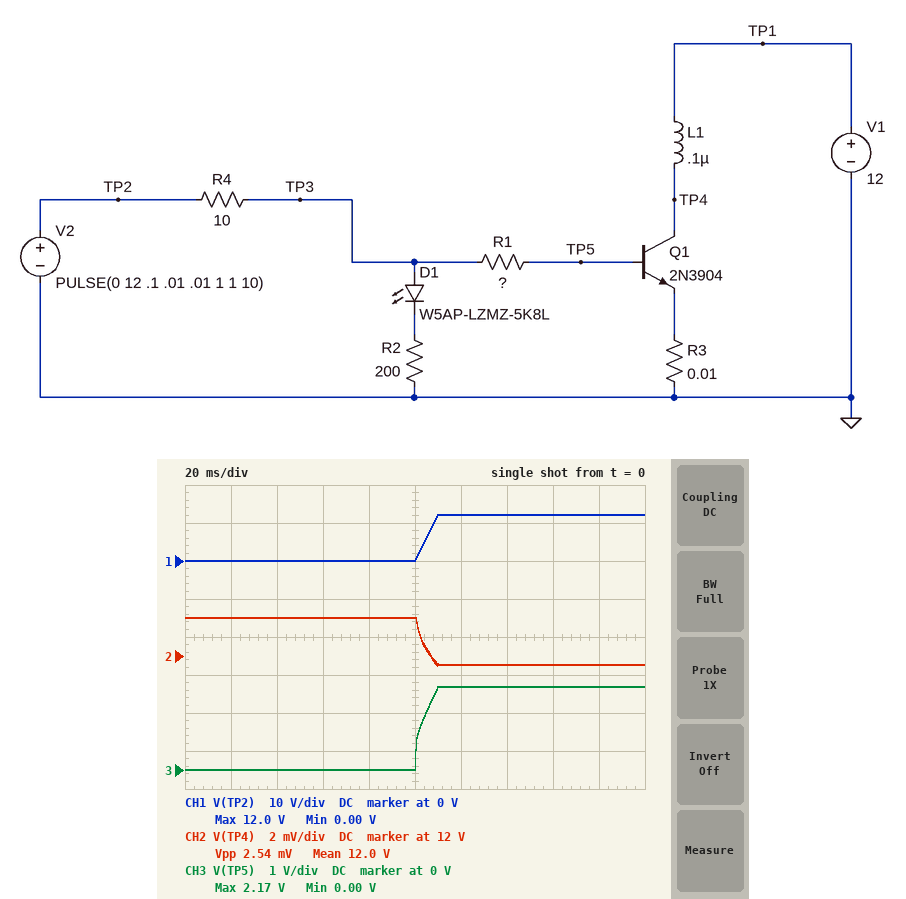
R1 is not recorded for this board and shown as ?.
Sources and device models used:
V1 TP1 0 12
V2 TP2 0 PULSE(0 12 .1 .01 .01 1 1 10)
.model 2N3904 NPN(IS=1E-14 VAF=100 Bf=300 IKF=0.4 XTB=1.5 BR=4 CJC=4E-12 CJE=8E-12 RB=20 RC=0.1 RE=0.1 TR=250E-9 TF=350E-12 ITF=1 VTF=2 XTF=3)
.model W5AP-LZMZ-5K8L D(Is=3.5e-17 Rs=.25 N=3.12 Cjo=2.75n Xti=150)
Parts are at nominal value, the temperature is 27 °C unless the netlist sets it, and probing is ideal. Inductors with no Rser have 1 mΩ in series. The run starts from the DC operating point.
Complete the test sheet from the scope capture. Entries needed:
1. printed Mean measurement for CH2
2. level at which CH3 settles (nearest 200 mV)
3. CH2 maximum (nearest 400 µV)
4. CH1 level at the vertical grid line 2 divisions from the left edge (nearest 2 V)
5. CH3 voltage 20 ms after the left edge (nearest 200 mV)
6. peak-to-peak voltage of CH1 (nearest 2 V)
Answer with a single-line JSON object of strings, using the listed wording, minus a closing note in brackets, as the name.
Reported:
{"printed Mean measurement for CH2": "12.0 V", "level at which CH3 settles": "2.2 V", "CH2 maximum": "12.0000 V", "CH1 level at the vertical grid line 2 divisions from the left edge": "0 V", "CH3 voltage 20 ms after the left edge": "0 V", "peak-to-peak voltage of CH1": "12 V"}
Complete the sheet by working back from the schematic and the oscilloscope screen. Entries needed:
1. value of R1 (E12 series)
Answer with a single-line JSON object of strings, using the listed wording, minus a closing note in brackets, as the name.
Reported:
{"value of R1": "180 Ω"}
